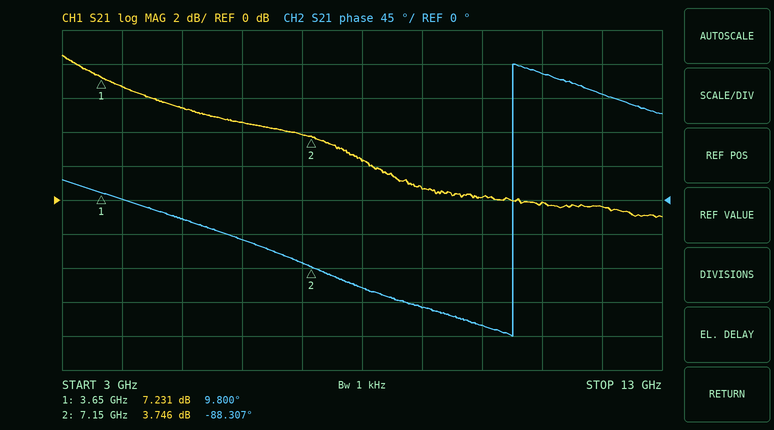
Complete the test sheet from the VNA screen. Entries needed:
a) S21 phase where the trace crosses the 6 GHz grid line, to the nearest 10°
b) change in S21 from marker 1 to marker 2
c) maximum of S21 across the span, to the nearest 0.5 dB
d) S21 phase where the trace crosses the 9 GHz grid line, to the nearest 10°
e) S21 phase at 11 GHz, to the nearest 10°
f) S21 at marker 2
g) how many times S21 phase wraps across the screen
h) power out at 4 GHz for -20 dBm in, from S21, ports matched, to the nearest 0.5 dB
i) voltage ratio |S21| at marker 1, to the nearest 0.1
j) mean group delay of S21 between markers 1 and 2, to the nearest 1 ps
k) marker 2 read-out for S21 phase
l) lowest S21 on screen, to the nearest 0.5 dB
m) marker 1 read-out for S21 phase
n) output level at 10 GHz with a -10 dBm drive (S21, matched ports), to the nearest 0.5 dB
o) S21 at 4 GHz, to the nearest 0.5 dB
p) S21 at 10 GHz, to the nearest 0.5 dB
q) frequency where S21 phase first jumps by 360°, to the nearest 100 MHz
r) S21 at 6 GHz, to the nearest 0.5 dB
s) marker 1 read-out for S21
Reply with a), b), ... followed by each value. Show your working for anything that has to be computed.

a) -50°
b) 3.746 − (7.231) = -3.485 dB
c) 8.5 dB
d) -140°
e) 170°
f) 3.746 dB
g) 1
h) -20 dBm + (6.5 dB) = -13.5 dBm
i) 10^(7.231/20) ≈ 2.3
j) −(-88.307° − (9.8°))/(360° × 3.5 GHz) ≈ 78 ps
k) -88.307°
l) -1.0 dB
m) 9.800°
n) -10 dBm + (0.0 dB) = -10.0 dBm
o) 6.5 dB
p) 0.0 dB
q) 10.5 GHz
r) 4.5 dB
s) 7.231 dB
